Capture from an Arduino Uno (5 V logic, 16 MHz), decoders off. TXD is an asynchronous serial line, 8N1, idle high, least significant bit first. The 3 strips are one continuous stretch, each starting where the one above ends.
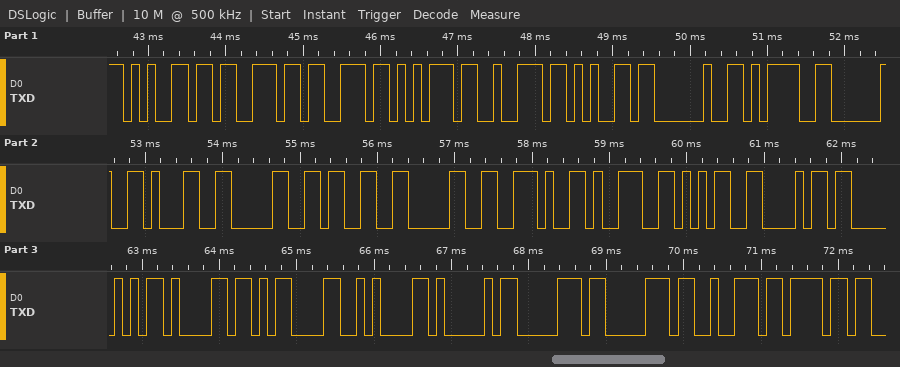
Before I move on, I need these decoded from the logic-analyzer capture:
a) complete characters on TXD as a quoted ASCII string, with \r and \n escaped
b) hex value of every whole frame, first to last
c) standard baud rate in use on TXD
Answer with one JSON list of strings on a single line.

["\"essure = 1030.95hPa\\r\\nAppro\"", "65 73 73 75 72 65 20 3D 20 31 30 33 30 2E 39 35 68 50 61 0D 0A 41 70 70 72 6F", "9600 baud"]
